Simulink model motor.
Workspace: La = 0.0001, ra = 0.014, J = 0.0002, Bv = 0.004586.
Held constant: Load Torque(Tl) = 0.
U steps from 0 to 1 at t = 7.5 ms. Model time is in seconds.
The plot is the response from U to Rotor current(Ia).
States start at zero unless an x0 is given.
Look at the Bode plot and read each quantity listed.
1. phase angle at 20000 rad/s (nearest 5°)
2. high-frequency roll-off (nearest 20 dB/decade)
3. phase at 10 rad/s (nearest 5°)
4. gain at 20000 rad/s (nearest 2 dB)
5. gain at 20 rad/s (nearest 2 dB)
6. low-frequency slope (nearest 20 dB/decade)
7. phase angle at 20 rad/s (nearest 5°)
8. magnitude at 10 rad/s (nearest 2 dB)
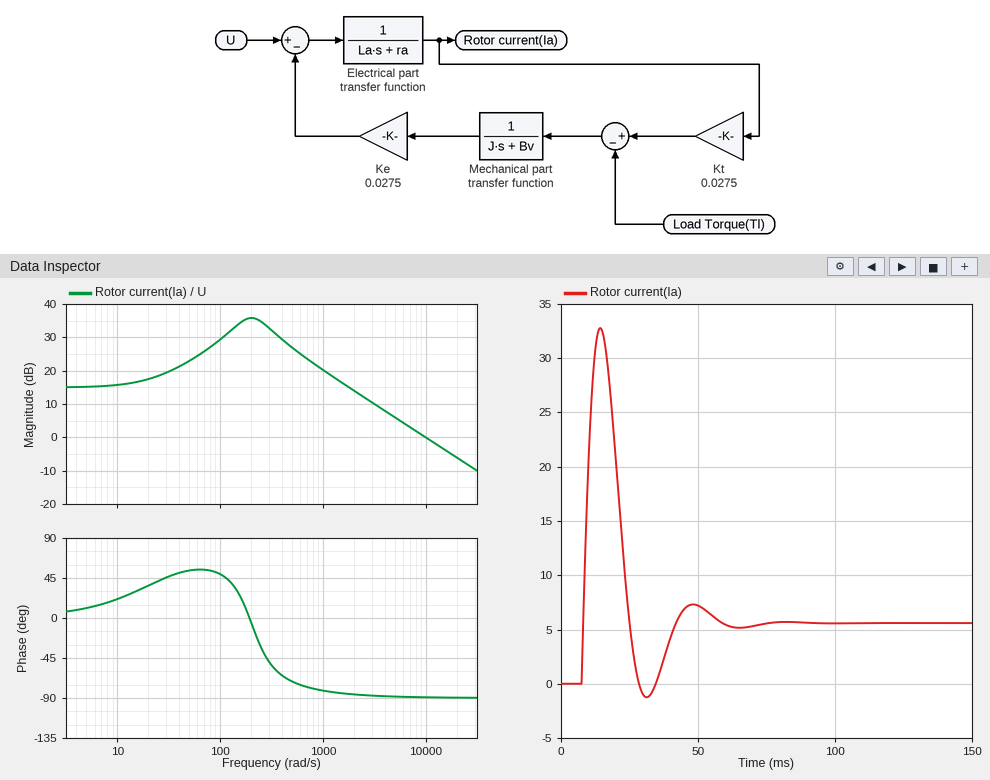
-90°
-20 dB/decade
20°
-6 dB
18 dB
0 dB/decade
35°
16 dB
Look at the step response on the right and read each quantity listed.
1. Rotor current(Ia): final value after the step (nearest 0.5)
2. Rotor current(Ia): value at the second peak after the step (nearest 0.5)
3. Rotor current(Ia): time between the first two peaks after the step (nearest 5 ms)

5.5
7.5
35 ms
